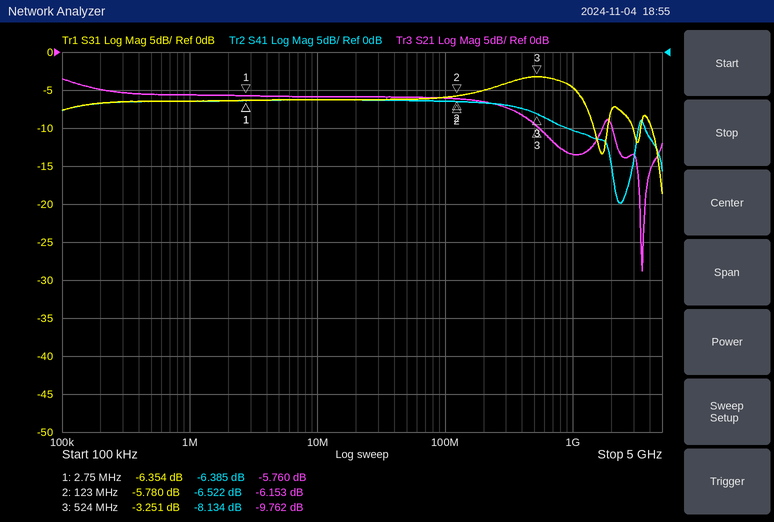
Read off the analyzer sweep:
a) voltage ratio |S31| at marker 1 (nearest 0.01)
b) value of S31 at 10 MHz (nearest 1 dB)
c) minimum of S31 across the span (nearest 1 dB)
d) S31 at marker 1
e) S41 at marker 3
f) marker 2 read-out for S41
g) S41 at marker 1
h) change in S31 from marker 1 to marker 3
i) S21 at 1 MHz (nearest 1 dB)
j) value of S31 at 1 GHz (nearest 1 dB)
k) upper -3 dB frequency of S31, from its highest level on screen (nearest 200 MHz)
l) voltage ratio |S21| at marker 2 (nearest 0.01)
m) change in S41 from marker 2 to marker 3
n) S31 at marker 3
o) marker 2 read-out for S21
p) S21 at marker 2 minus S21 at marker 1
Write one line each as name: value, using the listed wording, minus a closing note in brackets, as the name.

voltage ratio |S31| at marker 1: 0.48
value of S31 at 10 MHz: -6 dB
minimum of S31 across the span: -19 dB
S31 at marker 1: -6.354 dB
S41 at marker 3: -8.134 dB
marker 2 read-out for S41: -6.522 dB
S41 at marker 1: -6.385 dB
change in S31 from marker 1 to marker 3: 3.103 dB
S21 at 1 MHz: -6 dB
value of S31 at 1 GHz: -5 dB
upper -3 dB frequency of S31, from its highest level on screen: 1.2 GHz
voltage ratio |S21| at marker 2: 0.49
change in S41 from marker 2 to marker 3: -1.612 dB
S31 at marker 3: -3.251 dB
marker 2 read-out for S21: -6.153 dB
S21 at marker 2 minus S21 at marker 1: -0.393 dB
